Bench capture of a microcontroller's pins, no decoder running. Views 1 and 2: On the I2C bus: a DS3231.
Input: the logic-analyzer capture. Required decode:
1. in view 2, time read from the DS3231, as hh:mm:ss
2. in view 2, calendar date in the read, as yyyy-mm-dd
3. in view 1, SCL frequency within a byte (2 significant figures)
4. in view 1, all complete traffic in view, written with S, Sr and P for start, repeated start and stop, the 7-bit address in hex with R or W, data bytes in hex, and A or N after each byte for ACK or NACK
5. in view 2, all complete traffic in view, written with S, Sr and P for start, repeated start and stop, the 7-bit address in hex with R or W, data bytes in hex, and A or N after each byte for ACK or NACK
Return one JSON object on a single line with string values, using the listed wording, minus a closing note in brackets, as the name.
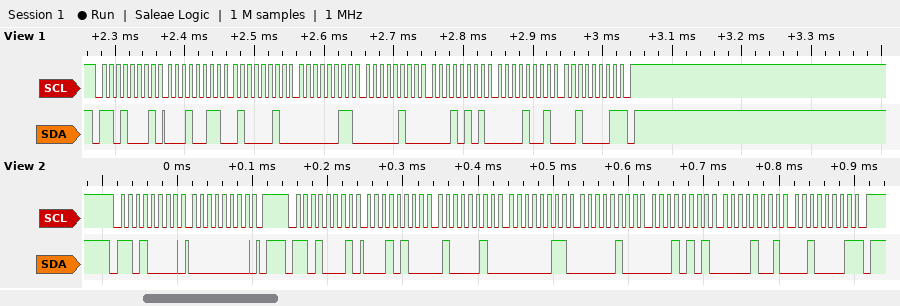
{"in view 2, time read from the DS3231, as hh:mm:ss": "03:42:14", "in view 2, calendar date in the read, as yyyy-mm-dd": "2021-09-15", "in view 1, SCL frequency within a byte": "100 kHz", "in view 1, all complete traffic in view, written with S, Sr and P for start, repeated start and stop, the 7-bit address in hex with R or W, data bytes in hex, and A or N after each byte for ACK or NACK": "S 68R A 13 A 42 A 03 A 04 A 15 A 09 A 21 N P", "in view 2, all complete traffic in view, written with S, Sr and P for start, repeated start and stop, the 7-bit address in hex with R or W, data bytes in hex, and A or N after each byte for ACK or NACK": "S 68W A 00 A P S 68R A 14 A 42 A 03 A 04 A 15 A 09 A 21 N P"}
